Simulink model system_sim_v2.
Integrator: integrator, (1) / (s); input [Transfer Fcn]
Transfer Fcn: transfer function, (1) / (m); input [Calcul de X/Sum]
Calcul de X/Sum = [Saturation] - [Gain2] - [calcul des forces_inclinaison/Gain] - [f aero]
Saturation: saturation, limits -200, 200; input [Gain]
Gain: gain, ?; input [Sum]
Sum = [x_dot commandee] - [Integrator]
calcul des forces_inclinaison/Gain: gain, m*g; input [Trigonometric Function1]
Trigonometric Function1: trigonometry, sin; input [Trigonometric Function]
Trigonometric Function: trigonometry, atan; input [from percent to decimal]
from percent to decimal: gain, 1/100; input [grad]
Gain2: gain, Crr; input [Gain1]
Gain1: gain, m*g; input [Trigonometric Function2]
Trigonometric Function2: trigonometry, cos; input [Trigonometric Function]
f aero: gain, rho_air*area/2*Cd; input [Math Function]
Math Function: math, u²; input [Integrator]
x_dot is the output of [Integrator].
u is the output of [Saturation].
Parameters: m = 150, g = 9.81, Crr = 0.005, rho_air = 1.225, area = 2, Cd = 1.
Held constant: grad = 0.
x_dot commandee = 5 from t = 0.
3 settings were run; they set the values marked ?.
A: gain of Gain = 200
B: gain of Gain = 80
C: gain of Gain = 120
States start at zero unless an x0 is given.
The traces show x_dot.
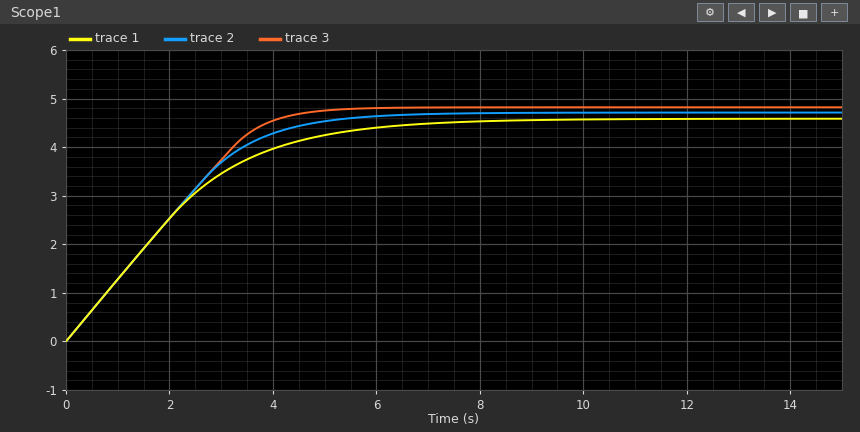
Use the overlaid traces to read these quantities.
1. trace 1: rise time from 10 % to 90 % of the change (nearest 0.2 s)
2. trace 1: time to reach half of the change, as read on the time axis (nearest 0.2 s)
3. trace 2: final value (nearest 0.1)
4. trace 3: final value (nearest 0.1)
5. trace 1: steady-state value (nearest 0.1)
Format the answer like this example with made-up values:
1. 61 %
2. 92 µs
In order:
1. 4.2 s
2. 1.8 s
3. 4.7
4. 4.8
5. 4.6
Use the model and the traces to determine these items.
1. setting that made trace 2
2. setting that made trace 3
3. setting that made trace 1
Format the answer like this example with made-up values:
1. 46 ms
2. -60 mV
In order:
1. C
2. A
3. B
